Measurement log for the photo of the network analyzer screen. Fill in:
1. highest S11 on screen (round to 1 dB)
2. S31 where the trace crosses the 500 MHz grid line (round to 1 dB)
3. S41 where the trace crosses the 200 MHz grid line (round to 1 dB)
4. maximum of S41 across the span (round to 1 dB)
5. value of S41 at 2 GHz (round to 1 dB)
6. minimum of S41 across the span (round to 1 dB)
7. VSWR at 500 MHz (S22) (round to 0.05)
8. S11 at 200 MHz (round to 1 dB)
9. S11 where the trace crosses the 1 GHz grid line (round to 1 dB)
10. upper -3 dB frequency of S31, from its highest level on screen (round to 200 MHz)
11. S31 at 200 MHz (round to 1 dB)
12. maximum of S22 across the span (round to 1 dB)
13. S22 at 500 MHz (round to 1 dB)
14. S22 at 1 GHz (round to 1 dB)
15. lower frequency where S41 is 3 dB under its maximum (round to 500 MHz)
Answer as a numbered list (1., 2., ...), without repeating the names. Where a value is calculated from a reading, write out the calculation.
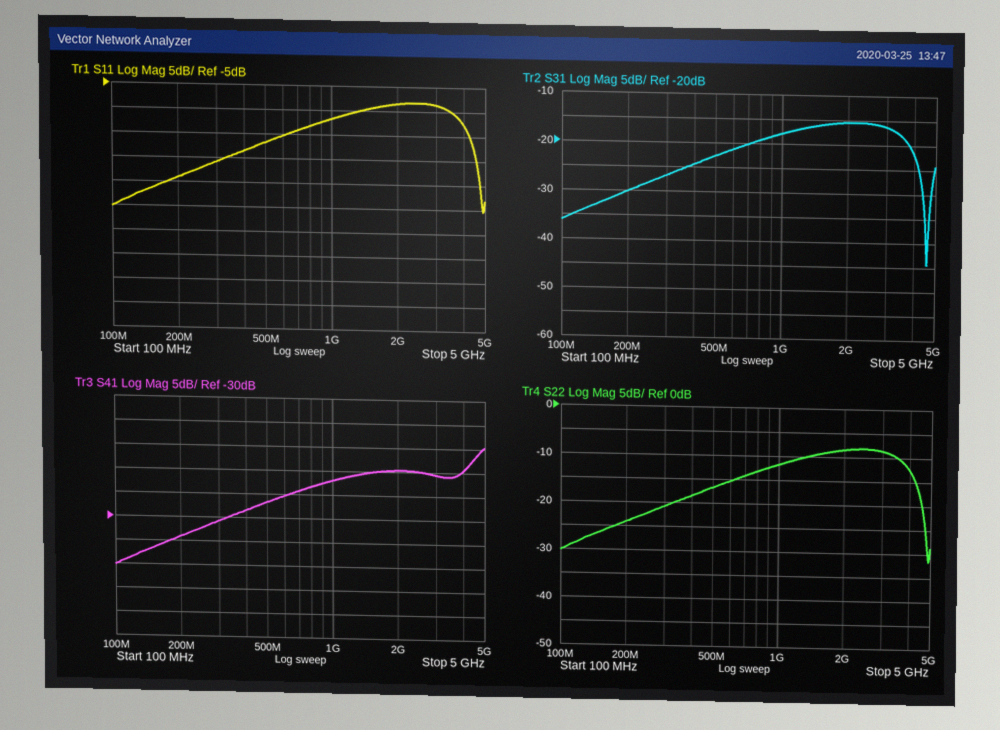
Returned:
1. -8 dB
2. -23 dB
3. -34 dB
4. -15 dB
5. -20 dB
6. -40 dB
7. |Γ| = 10^(-17/20) = 0.1413; VSWR = (1 + 0.1413)/(1 − 0.1413) ≈ 1.33, so 1.35 to the nearest 0.05
8. -24 dB
9. -12 dB
10. 3.6 GHz
11. -30 dB
12. -8 dB
13. -17 dB
14. -12 dB
15. 4.5 GHz
